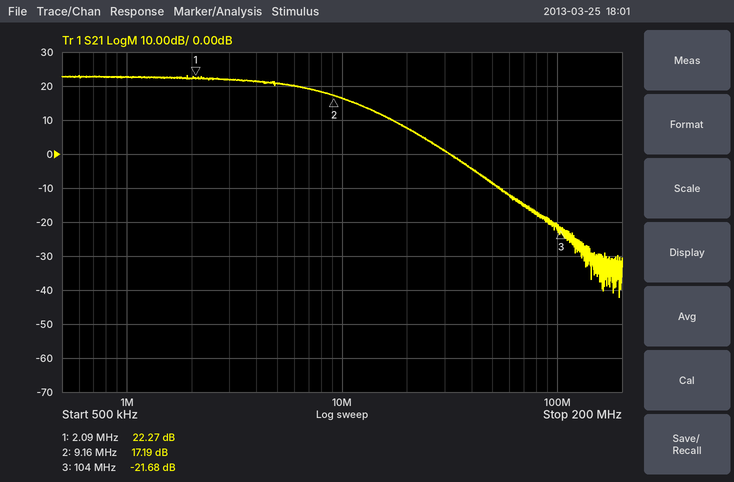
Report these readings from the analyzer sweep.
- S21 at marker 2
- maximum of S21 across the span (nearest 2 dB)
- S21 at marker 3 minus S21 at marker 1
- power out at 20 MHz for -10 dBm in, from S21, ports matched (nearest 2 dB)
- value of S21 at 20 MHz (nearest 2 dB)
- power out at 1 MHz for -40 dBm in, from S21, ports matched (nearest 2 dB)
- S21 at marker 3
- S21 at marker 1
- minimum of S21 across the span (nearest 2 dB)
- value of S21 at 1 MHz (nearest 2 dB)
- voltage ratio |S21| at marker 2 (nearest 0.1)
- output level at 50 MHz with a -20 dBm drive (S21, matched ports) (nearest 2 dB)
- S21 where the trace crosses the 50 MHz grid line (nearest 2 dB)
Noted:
17.19 dB
24 dB
-43.95 dB
-2 dBm
8 dB
-18 dBm
-21.68 dB
22.27 dB
-42 dB
22 dB
7.2
-28 dBm
-8 dB
